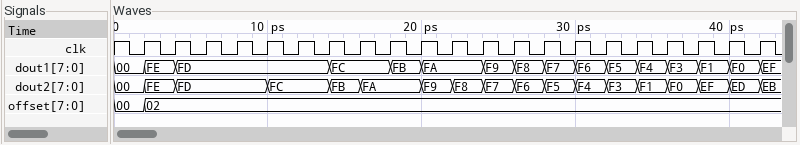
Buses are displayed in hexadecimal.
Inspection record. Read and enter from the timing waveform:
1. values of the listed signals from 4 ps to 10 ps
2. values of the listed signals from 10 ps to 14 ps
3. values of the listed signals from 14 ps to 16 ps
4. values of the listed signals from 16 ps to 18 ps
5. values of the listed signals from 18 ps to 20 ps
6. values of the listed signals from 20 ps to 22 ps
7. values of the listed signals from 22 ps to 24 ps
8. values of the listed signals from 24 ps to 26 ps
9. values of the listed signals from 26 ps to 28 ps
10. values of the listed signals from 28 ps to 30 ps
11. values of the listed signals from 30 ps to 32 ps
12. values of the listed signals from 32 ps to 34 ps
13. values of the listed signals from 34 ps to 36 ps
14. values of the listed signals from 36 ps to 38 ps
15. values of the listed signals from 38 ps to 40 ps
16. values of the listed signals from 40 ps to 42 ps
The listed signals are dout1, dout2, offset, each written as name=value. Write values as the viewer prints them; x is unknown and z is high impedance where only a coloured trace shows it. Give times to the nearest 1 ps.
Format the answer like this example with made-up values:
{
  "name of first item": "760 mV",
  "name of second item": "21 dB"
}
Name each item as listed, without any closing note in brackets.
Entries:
{
  "values of the listed signals from 4 ps to 10 ps": "dout1=FD, dout2=FD, offset=02",
  "values of the listed signals from 10 ps to 14 ps": "dout1=FD, dout2=FC, offset=02",
  "values of the listed signals from 14 ps to 16 ps": "dout1=FC, dout2=FB, offset=02",
  "values of the listed signals from 16 ps to 18 ps": "dout1=FC, dout2=FA, offset=02",
  "values of the listed signals from 18 ps to 20 ps": "dout1=FB, dout2=FA, offset=02",
  "values of the listed signals from 20 ps to 22 ps": "dout1=FA, dout2=F9, offset=02",
  "values of the listed signals from 22 ps to 24 ps": "dout1=FA, dout2=F8, offset=02",
  "values of the listed signals from 24 ps to 26 ps": "dout1=F9, dout2=F7, offset=02",
  "values of the listed signals from 26 ps to 28 ps": "dout1=F8, dout2=F6, offset=02",
  "values of the listed signals from 28 ps to 30 ps": "dout1=F7, dout2=F5, offset=02",
  "values of the listed signals from 30 ps to 32 ps": "dout1=F6, dout2=F4, offset=02",
  "values of the listed signals from 32 ps to 34 ps": "dout1=F5, dout2=F3, offset=02",
  "values of the listed signals from 34 ps to 36 ps": "dout1=F4, dout2=F1, offset=02",
  "values of the listed signals from 36 ps to 38 ps": "dout1=F3, dout2=F0, offset=02",
  "values of the listed signals from 38 ps to 40 ps": "dout1=F1, dout2=EF, offset=02",
  "values of the listed signals from 40 ps to 42 ps": "dout1=F0, dout2=ED, offset=02"
}
